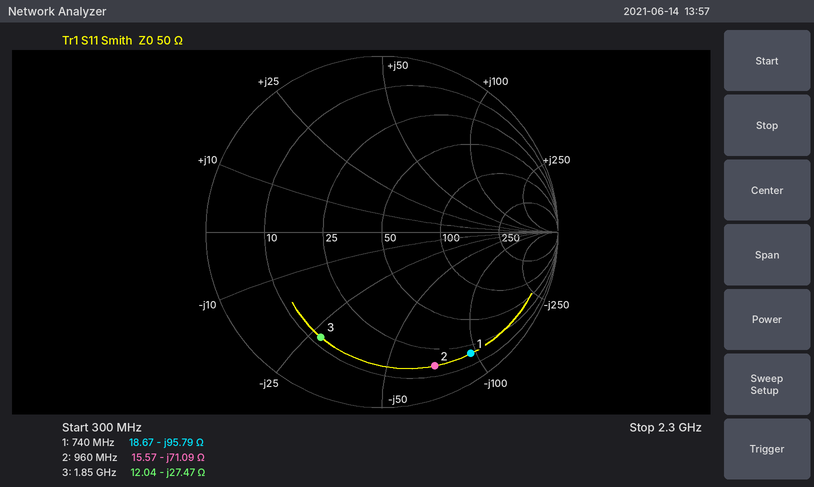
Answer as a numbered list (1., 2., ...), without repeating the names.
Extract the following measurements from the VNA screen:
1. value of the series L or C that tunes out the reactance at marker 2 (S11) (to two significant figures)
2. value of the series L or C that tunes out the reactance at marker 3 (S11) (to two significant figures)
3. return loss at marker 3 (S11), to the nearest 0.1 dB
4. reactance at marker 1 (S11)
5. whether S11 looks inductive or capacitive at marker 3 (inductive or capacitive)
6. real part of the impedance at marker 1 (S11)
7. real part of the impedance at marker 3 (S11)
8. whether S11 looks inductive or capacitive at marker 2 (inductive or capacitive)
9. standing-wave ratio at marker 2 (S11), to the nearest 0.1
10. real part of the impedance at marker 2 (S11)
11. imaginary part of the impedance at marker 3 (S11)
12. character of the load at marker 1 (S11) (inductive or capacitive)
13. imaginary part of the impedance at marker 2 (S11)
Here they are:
1. 12 nH
2. 2.4 nH
3. 3.2 dB
4. -95.79 Ω
5. capacitive
6. 18.67 Ω
7. 12.04 Ω
8. capacitive
9. 9.9
10. 15.57 Ω
11. -27.47 Ω
12. capacitive
13. -71.09 Ω
